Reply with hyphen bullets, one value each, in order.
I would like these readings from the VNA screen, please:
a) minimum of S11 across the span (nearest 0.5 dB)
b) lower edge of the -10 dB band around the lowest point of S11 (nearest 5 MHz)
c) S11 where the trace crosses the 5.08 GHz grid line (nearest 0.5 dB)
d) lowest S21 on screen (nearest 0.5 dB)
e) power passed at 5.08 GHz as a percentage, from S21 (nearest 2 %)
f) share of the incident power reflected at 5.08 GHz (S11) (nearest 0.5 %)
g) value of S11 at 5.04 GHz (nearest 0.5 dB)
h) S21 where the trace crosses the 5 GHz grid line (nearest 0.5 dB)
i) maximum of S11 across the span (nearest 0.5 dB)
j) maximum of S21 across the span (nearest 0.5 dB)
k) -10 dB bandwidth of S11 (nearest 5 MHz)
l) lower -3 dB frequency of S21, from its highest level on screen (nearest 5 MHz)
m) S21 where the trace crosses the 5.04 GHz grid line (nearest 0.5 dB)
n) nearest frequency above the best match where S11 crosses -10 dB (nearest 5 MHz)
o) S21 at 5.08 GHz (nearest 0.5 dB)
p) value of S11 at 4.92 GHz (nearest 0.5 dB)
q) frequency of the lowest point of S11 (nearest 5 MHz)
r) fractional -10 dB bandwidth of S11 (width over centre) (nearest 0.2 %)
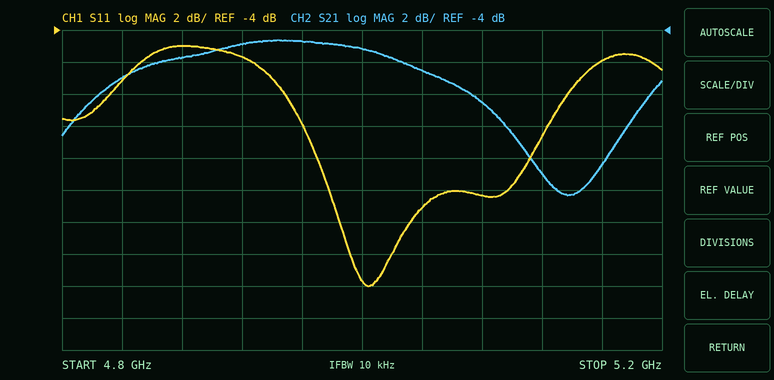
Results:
- -20.0 dB
- 4.960 GHz
- -14.5 dB
- -14.5 dB
- 14 %
- 3.5 %
- -15.0 dB
- -5.0 dB
- -5.0 dB
- -4.5 dB
- 165 MHz
- 4.830 GHz
- -6.5 dB
- 5.125 GHz
- -8.5 dB
- -5.5 dB
- 5.005 GHz
- 3.2 %
